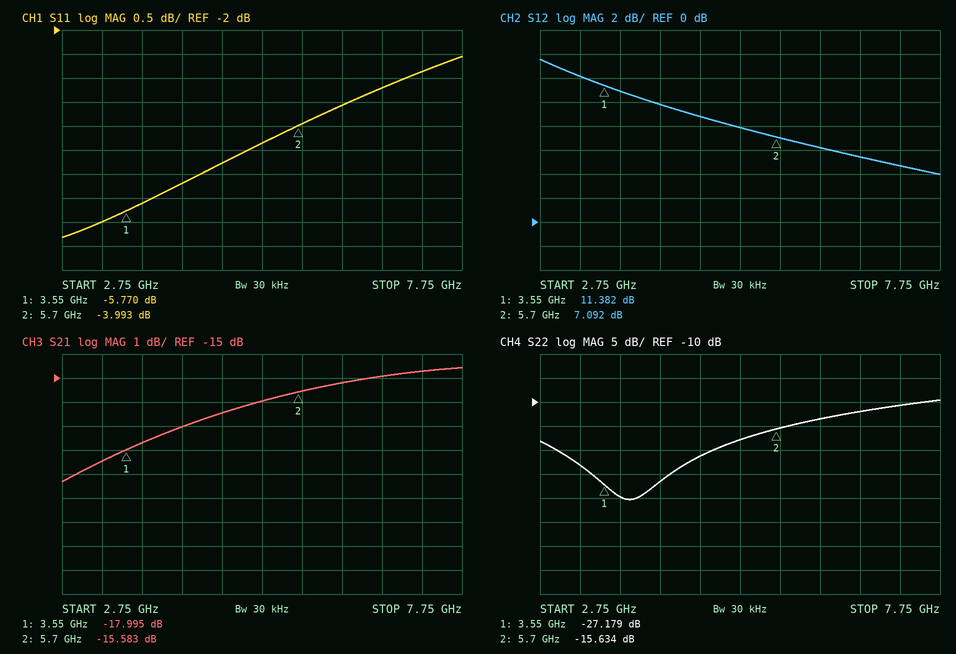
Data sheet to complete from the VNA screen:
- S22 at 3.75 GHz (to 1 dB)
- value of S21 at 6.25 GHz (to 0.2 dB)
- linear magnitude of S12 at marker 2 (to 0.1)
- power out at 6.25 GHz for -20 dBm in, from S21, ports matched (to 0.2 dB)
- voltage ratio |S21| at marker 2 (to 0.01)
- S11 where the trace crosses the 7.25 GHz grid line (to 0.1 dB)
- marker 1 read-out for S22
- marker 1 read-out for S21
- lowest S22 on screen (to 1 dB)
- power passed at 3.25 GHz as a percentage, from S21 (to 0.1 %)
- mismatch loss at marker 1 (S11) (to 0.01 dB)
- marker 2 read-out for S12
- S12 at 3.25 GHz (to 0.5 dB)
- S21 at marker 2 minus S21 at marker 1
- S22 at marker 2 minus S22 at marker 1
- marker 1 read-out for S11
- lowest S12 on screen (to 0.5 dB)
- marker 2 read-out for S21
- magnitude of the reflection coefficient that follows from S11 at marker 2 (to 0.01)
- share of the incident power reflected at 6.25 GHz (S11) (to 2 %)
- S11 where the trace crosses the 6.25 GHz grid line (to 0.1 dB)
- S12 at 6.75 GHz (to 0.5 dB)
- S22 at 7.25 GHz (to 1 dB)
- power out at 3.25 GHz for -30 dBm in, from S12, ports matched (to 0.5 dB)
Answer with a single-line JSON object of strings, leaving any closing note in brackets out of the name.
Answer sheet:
{"S22 at 3.75 GHz": "-30 dB", "value of S21 at 6.25 GHz": "-15.2 dB", "linear magnitude of S12 at marker 2": "2.3", "power out at 6.25 GHz for -20 dBm in, from S21, ports matched": "-35.2 dBm", "voltage ratio |S21| at marker 2": "0.17", "S11 where the trace crosses the 7.25 GHz grid line": "-2.9 dB", "marker 1 read-out for S22": "-27.179 dB", "marker 1 read-out for S21": "-17.995 dB", "lowest S22 on screen": "-30 dB", "power passed at 3.25 GHz as a percentage, from S21": "1.4 %", "mismatch loss at marker 1 (S11)": "1.34 dB", "marker 2 read-out for S12": "7.092 dB", "S12 at 3.25 GHz": "12.0 dB", "S21 at marker 2 minus S21 at marker 1": "2.412 dB", "S22 at marker 2 minus S22 at marker 1": "11.545 dB", "marker 1 read-out for S11": "-5.770 dB", "lowest S12 on screen": "4.0 dB", "marker 2 read-out for S21": "-15.583 dB", "magnitude of the reflection coefficient that follows from S11 at marker 2": "0.63", "share of the incident power reflected at 6.25 GHz (S11)": "44 %", "S11 where the trace crosses the 6.25 GHz grid line": "-3.6 dB", "S12 at 6.75 GHz": "5.5 dB", "S22 at 7.25 GHz": "-11 dB", "power out at 3.25 GHz for -30 dBm in, from S12, ports matched": "-18.0 dBm"}
